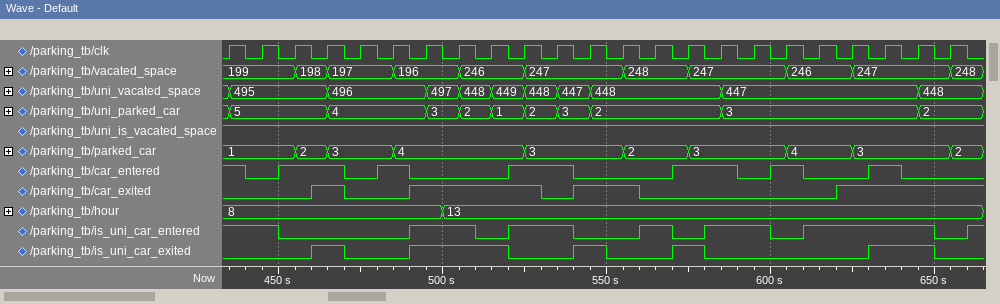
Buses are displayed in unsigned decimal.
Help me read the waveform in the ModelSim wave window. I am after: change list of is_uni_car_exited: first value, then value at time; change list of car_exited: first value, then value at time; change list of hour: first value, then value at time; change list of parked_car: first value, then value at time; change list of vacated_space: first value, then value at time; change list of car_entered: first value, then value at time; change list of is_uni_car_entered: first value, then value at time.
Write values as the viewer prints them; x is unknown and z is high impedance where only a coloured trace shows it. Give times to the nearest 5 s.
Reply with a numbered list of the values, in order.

1. 0, 1 at 460 s, 0 at 470 s, 1 at 490 s, 0 at 520 s, 1 at 540 s, 0 at 550 s, 1 at 570 s, 0 at 580 s, 1 at 630 s, 0 at 650 s
2. 0, 1 at 460 s, 0 at 470 s, 1 at 490 s, 0 at 530 s, 1 at 540 s, 0 at 560 s, 1 at 620 s
3. 8, 13 at 500 s
4. 1, 2 at 455 s, 3 at 465 s, 4 at 485 s, 3 at 525 s, 2 at 555 s, 3 at 575 s, 4 at 605 s, 3 at 625 s, 2 at 655 s
5. 199, 198 at 455 s, 197 at 465 s, 196 at 485 s, 246 at 505 s, 247 at 525 s, 248 at 555 s, 247 at 575 s, 246 at 605 s, 247 at 625 s, 248 at 655 s
6. 1, 0 at 440 s, 1 at 450 s, 0 at 470 s, 1 at 480 s, 0 at 490 s, 1 at 520 s, 0 at 540 s, 1 at 570 s, 0 at 590 s, 1 at 600 s, 0 at 610 s, 1 at 630 s, 0 at 640 s
7. 1, 0 at 450 s, 1 at 490 s, 0 at 510 s, 1 at 520 s, 0 at 540 s, 1 at 560 s, 0 at 570 s, 1 at 580 s, 0 at 600 s, 1 at 610 s, 0 at 650 s, 1 at 660 s
